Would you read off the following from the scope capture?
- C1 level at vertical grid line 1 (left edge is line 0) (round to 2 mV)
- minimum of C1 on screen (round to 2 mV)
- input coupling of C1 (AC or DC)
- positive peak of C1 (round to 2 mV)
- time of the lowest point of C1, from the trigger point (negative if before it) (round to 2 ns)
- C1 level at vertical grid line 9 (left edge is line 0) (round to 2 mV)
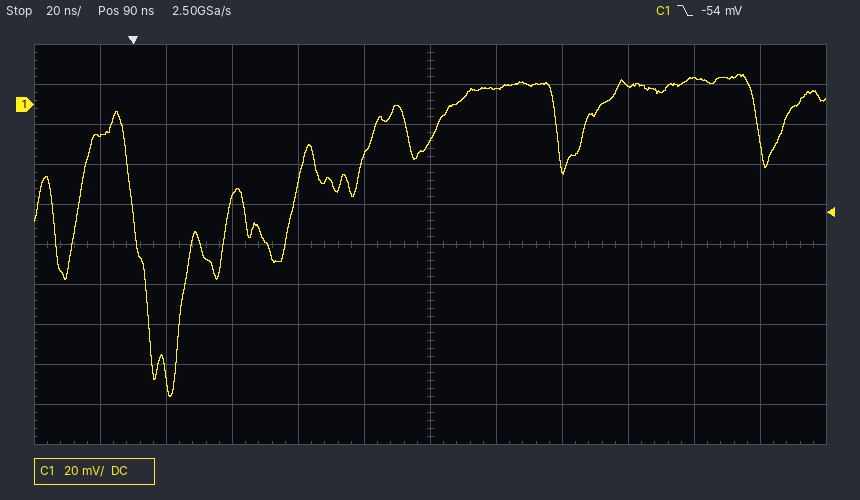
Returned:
-16 mV
-146 mV
DC
16 mV
+12 ns
10 mV
